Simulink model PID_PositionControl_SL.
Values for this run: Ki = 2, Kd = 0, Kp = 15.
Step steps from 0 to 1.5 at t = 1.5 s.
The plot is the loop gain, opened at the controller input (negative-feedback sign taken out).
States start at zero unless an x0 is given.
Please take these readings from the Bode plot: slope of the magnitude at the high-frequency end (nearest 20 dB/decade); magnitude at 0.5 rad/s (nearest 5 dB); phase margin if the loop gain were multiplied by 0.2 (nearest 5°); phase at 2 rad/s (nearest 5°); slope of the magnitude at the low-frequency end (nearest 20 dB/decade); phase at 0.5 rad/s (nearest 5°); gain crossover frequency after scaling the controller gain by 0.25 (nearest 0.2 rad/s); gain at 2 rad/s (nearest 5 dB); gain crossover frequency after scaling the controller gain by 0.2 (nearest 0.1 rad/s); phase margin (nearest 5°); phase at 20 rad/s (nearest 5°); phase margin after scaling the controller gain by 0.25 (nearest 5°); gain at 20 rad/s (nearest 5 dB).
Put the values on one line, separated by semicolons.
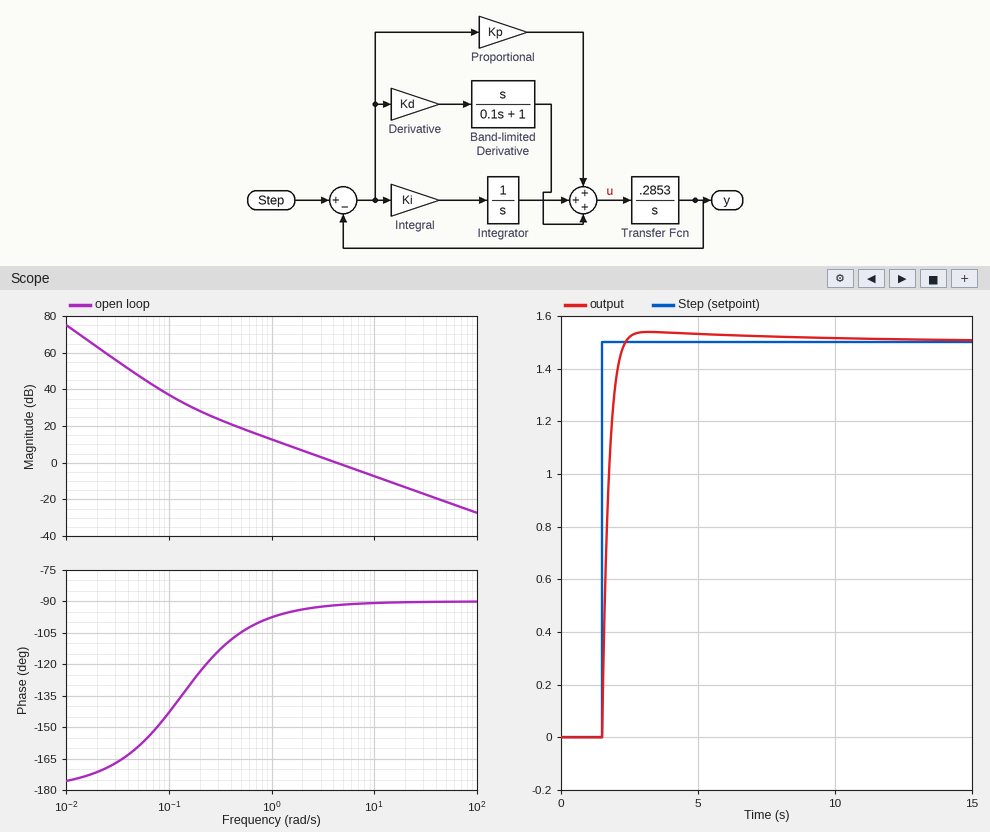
-20 dB/decade; 20 dB; 80°; -95°; -40 dB/decade; -105°; 1.0 rad/s; 5 dB; 0.9 rad/s; 90°; -90°; 85°; -15 dB
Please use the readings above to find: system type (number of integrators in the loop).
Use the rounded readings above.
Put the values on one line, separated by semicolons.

2
